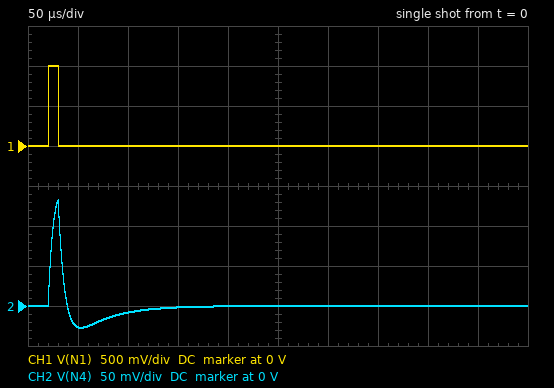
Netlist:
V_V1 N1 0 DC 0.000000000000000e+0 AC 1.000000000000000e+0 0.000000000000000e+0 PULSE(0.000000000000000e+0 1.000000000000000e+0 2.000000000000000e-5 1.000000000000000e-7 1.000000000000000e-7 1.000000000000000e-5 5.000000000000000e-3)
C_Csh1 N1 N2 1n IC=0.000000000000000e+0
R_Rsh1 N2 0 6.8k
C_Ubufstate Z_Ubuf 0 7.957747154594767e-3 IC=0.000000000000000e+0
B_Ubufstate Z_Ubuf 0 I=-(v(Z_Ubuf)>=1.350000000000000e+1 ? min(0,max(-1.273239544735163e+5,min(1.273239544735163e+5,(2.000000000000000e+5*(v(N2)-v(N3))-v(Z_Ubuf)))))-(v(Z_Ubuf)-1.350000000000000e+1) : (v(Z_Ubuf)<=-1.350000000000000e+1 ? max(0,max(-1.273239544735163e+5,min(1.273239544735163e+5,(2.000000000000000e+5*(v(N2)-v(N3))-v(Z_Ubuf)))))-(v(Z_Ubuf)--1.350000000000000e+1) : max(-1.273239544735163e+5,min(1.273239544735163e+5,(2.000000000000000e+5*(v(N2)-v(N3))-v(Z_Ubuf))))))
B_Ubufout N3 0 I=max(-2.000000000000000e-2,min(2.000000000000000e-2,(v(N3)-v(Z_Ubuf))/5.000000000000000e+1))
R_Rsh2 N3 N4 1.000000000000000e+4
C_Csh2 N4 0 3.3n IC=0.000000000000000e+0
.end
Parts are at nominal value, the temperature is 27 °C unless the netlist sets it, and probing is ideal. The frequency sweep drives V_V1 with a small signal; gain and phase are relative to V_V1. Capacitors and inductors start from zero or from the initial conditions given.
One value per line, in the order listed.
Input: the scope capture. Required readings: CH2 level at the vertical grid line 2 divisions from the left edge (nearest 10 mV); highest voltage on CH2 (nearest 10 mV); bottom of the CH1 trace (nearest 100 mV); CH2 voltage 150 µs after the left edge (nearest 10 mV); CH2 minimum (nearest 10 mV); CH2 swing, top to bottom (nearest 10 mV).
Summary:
-10 mV
130 mV
0 V
0 V
-30 mV
160 mV
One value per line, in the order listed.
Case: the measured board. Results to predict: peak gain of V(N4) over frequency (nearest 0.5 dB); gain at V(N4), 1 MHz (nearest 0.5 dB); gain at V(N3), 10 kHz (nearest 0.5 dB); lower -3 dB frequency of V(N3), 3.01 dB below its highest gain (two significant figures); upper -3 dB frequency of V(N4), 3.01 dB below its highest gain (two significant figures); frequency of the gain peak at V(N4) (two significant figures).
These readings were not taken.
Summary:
-15.5 dB
-46.5 dB
-8.0 dB
23 kHz
32 kHz
11 kHz
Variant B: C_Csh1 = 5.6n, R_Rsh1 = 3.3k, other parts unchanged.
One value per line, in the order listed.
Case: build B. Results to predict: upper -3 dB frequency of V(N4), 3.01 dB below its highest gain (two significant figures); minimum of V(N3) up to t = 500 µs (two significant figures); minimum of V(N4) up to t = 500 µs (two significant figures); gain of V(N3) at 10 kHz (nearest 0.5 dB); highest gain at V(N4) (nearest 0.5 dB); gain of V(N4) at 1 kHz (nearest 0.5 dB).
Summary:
16 kHz
-420 mV
-39 mV
-2.5 dB
-9.0 dB
-19.0 dB
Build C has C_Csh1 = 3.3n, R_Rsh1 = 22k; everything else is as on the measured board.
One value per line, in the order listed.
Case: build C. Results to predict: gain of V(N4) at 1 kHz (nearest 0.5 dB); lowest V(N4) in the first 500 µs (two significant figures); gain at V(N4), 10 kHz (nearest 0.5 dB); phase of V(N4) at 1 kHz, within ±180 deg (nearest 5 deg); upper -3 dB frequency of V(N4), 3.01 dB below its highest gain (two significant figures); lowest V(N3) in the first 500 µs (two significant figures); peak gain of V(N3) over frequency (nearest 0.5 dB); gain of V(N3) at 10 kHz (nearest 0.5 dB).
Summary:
-8.0 dB
-37 mV
-7.5 dB
55 deg
8.3 kHz
-130 mV
0 dB
0 dB
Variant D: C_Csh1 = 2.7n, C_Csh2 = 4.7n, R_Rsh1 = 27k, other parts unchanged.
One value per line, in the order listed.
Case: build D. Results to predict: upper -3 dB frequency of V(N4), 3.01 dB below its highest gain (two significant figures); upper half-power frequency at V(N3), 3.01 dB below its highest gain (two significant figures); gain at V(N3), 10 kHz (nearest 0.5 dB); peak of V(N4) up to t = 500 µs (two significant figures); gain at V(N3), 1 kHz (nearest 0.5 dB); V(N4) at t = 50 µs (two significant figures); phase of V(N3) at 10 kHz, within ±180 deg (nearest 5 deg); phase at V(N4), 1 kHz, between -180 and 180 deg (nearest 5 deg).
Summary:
6.7 kHz
4.0 MHz
0 dB
180 mV
-7.5 dB
80 mV
10 deg
50 deg
